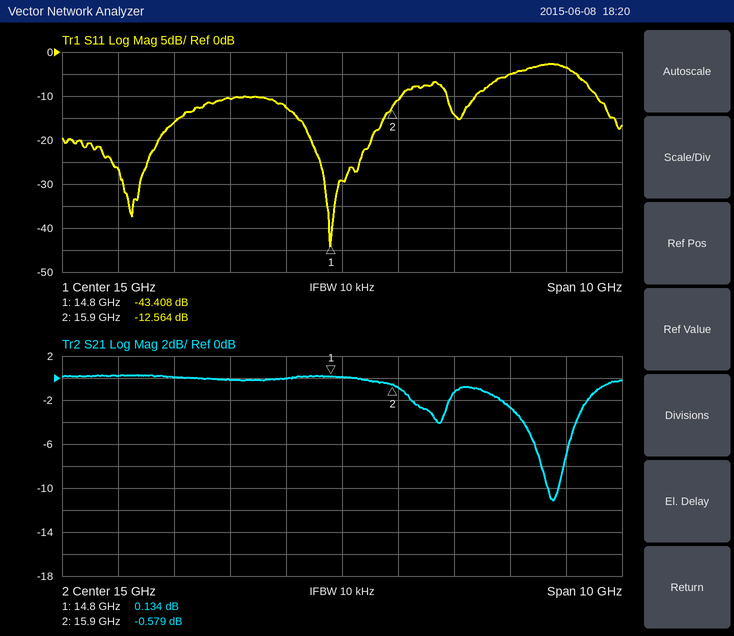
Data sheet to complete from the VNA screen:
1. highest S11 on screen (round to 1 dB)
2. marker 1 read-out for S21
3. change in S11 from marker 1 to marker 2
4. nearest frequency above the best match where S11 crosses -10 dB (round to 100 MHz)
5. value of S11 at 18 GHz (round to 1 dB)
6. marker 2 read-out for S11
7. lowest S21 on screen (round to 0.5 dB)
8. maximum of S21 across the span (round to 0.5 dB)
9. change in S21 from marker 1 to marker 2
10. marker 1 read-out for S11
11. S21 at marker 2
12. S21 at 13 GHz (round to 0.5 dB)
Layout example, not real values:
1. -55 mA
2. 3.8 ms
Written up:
1. -3 dB
2. 0.134 dB
3. 30.844 dB
4. 16.1 GHz
5. -5 dB
6. -12.564 dB
7. -11.0 dB
8. 0.5 dB
9. -0.713 dB
10. -43.408 dB
11. -0.579 dB
12. 0.0 dB
